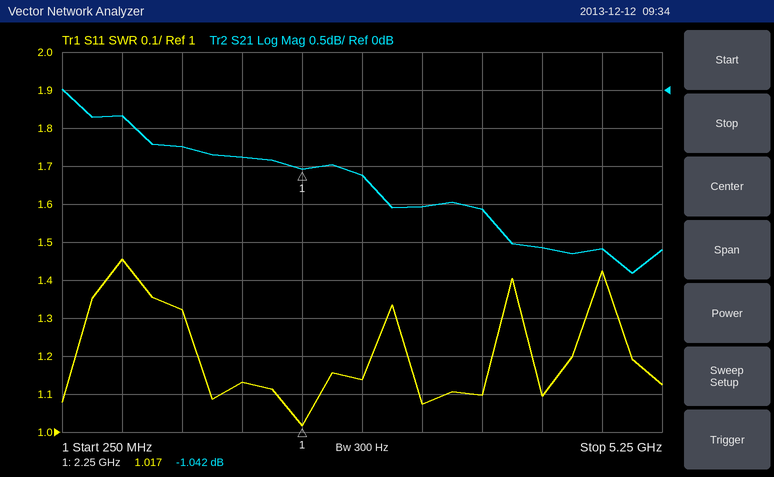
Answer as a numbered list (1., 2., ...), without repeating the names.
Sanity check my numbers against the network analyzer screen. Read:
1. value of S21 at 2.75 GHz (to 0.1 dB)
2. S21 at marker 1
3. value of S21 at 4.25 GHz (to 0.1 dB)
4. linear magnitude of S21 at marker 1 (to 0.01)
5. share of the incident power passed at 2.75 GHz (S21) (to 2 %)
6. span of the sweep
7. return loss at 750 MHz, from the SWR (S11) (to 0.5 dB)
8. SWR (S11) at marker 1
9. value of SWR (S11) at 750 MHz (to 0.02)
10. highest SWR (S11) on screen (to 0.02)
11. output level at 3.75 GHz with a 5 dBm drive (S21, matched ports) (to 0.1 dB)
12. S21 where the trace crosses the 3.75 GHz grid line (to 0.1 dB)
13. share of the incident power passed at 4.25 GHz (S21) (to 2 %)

1. -1.1 dB
2. -1.042 dB
3. -2.1 dB
4. 0.89
5. 78 %
6. 5 GHz
7. 14.5 dB
8. 1.017
9. 1.46
10. 1.46
11. 3.4 dBm
12. -1.6 dB
13. 62 %
